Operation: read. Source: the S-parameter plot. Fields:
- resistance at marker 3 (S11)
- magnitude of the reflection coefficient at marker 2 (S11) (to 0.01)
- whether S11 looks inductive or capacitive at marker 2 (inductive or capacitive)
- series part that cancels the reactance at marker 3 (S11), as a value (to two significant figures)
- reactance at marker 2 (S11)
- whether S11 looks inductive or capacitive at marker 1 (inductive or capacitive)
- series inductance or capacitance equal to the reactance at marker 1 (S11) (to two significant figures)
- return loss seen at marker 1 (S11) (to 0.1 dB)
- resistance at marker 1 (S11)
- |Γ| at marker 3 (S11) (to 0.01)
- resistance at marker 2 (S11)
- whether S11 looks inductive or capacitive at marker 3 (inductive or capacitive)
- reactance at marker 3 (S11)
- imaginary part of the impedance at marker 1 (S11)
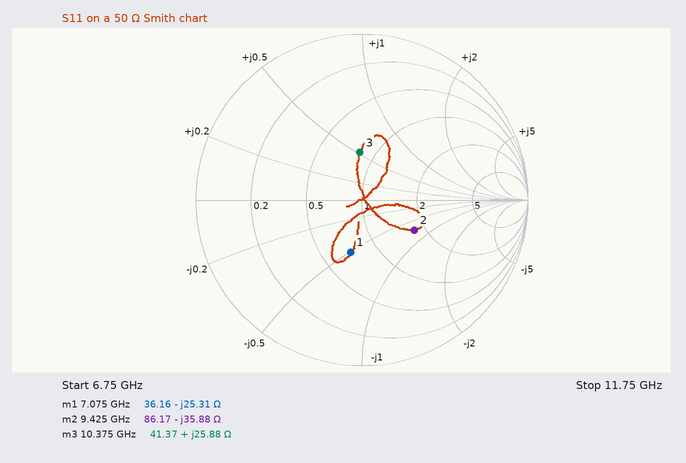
41.37 Ω
0.36
capacitive
590 fF
-35.88 Ω
capacitive
890 fF
9.9 dB
36.16 Ω
0.29
86.17 Ω
inductive
+25.88 Ω
-25.31 Ω
